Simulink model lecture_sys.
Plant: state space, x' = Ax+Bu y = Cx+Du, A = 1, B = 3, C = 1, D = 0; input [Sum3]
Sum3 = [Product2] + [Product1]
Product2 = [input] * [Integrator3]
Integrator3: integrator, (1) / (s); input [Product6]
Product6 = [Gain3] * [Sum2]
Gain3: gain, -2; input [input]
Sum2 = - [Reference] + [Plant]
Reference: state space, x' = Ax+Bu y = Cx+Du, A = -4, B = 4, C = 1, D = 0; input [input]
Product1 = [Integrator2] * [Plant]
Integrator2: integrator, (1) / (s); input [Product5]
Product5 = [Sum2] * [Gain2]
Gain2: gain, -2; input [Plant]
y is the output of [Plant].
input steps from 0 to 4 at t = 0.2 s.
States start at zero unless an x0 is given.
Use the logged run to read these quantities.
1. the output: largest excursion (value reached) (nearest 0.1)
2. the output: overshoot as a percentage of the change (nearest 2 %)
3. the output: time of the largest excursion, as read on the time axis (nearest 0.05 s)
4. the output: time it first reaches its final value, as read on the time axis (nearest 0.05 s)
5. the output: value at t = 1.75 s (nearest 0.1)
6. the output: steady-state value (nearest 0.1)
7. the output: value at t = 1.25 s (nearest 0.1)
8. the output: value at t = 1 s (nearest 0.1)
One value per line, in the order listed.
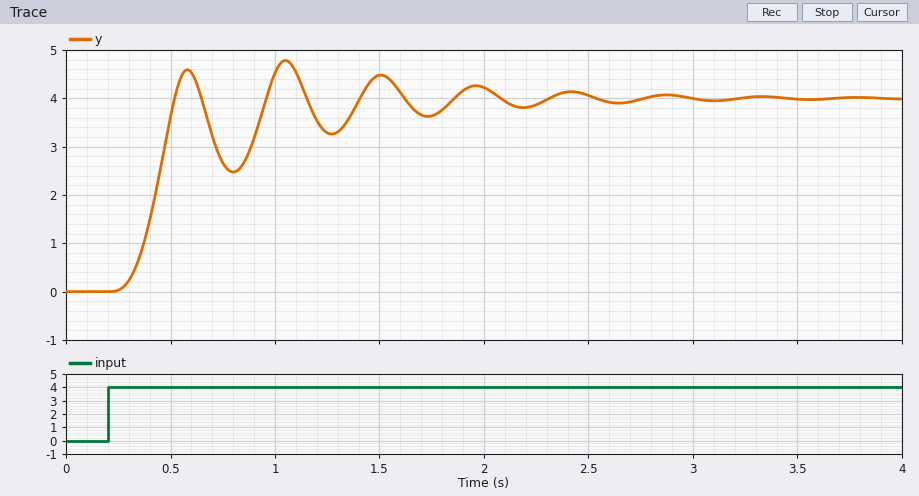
4.8
20 %
1.05 s
0.50 s
3.6
4.0
3.3
4.5
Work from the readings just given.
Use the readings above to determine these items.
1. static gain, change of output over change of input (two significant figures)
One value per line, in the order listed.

1.0
